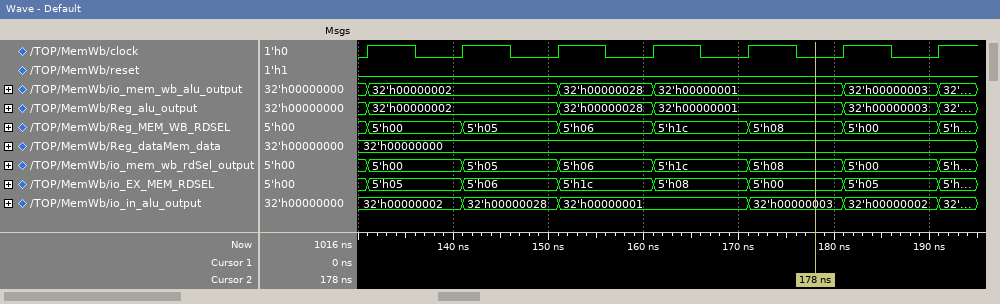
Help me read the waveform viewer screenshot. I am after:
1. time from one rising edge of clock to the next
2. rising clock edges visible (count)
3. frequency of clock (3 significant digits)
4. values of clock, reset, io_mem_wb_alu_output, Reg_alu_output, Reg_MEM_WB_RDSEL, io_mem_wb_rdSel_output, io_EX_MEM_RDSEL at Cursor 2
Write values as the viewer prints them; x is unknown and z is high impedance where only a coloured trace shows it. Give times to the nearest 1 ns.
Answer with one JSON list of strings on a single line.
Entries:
["10 ns", "7", "100 MHz", "clock=0, reset=0, io_mem_wb_alu_output=32'h00000001, Reg_alu_output=32'h00000001, Reg_MEM_WB_RDSEL=5'h08, io_mem_wb_rdSel_output=5'h08, io_EX_MEM_RDSEL=5'h00"]
